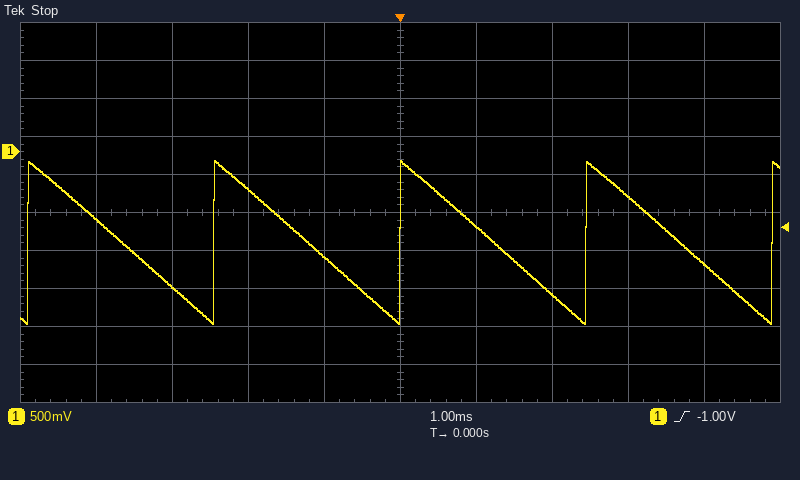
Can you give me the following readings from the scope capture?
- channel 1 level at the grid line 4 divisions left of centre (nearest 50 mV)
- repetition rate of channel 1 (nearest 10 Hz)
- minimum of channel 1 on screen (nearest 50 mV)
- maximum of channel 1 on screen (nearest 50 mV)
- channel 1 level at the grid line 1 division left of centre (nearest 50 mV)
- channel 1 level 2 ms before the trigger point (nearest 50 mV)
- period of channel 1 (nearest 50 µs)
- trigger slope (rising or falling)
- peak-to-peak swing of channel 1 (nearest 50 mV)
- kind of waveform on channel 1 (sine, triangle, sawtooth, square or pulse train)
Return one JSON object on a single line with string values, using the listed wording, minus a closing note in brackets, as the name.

{"channel 1 level at the grid line 4 divisions left of centre": "-900 mV", "repetition rate of channel 1": "410 Hz", "minimum of channel 1 on screen": "-2.25 V", "maximum of channel 1 on screen": "-100 mV", "channel 1 level at the grid line 1 division left of centre": "-1.40 V", "channel 1 level 2 ms before the trigger point": "-500 mV", "period of channel 1": "2.45 ms", "trigger slope": "rising", "peak-to-peak swing of channel 1": "2.15 V", "kind of waveform on channel 1": "sawtooth"}
